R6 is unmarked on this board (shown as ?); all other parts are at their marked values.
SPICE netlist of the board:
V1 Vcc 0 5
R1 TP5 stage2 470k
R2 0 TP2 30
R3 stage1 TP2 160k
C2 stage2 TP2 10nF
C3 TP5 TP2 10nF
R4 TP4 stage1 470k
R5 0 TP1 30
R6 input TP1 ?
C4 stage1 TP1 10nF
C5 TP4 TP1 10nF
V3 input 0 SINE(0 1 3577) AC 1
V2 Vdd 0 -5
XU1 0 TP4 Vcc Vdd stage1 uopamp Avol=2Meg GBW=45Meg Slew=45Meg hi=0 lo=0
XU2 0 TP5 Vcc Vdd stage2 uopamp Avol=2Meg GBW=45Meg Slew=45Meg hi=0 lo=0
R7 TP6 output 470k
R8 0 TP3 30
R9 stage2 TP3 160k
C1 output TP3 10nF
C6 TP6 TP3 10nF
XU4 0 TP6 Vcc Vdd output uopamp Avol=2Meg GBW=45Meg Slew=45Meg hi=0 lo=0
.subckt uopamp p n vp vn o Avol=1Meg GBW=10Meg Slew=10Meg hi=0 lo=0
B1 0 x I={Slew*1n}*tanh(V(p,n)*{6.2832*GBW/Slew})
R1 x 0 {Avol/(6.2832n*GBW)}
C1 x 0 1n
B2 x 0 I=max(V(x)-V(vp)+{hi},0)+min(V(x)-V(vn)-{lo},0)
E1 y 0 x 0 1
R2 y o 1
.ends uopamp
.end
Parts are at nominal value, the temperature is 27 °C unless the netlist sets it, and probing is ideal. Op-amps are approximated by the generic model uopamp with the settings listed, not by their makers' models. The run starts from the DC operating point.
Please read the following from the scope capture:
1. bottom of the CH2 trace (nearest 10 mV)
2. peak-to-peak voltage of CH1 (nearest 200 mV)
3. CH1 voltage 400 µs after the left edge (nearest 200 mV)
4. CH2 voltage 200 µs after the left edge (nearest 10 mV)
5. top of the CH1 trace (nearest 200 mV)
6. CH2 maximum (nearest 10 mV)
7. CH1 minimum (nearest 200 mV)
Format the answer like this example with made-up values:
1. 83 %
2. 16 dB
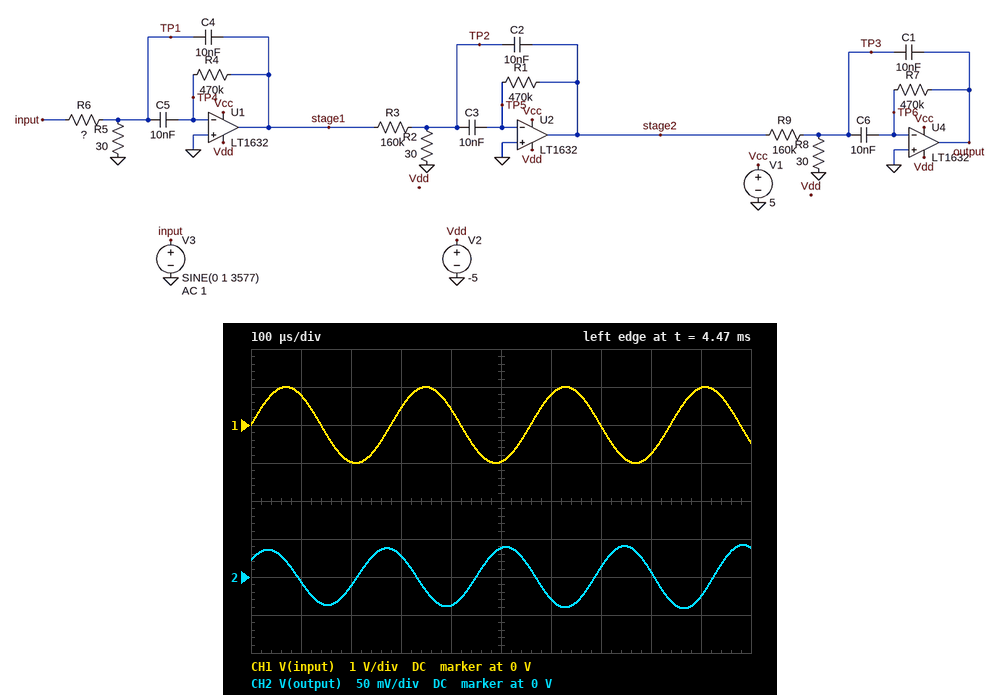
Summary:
1. -40 mV
2. 2.0 V
3. 400 mV
4. -10 mV
5. 1.0 V
6. 40 mV
7. -1.0 V
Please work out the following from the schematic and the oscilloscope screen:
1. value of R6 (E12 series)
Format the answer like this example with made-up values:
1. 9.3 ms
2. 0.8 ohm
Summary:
1. 120 kΩ
